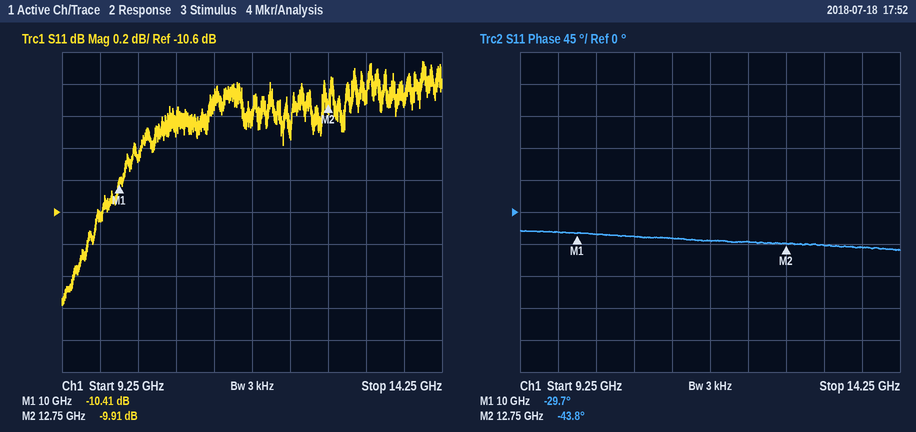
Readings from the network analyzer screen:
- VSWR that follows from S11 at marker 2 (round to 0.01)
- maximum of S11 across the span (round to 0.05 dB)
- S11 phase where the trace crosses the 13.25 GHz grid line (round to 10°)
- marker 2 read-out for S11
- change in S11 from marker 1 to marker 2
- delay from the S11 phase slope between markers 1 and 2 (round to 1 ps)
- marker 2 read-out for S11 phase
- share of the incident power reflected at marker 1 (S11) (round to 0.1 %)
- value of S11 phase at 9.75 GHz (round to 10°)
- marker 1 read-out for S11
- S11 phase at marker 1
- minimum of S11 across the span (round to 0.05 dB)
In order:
1.94
-9.65 dB
-50°
-9.91 dB
0.50 dB
14 ps
-43.8°
9.1 %
-30°
-10.41 dB
-29.7°
-11.20 dB
